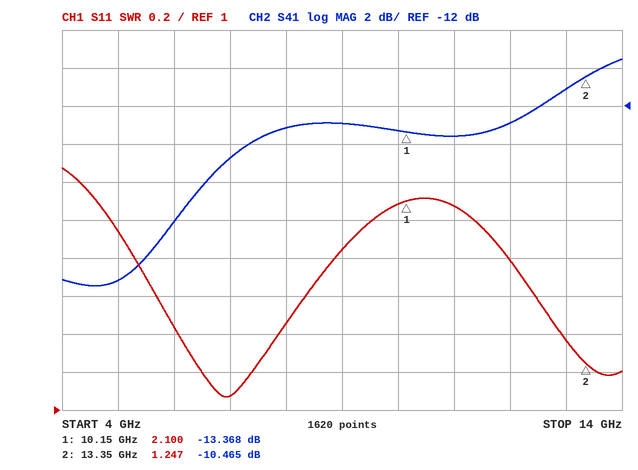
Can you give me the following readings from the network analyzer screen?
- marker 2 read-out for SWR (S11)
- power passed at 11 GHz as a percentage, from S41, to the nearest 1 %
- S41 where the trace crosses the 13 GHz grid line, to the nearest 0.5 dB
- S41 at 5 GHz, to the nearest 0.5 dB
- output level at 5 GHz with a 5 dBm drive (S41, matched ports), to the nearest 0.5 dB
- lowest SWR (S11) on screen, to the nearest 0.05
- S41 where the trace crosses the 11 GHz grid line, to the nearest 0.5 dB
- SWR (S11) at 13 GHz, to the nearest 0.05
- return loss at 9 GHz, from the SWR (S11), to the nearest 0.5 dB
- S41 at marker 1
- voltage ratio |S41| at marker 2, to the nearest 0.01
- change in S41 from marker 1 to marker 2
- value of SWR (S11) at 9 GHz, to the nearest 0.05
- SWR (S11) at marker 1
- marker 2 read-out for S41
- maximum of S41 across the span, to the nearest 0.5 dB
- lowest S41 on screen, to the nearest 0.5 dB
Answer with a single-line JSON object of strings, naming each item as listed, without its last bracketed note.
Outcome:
{"marker 2 read-out for SWR": "1.247", "power passed at 11 GHz as a percentage, from S41, to the nearest 1 %": "4 %", "S41 where the trace crosses the 13 GHz grid line, to the nearest 0.5 dB": "-11.0 dB", "S41 at 5 GHz, to the nearest 0.5 dB": "-21.0 dB", "output level at 5 GHz with a 5 dBm drive (S41, matched ports), to the nearest 0.5 dB": "-16.0 dBm", "lowest SWR (S11) on screen, to the nearest 0.05": "1.05", "S41 where the trace crosses the 11 GHz grid line, to the nearest 0.5 dB": "-13.5 dB", "SWR (S11) at 13 GHz, to the nearest 0.05": "1.35", "return loss at 9 GHz, from the SWR (S11), to the nearest 0.5 dB": "10.5 dB", "S41 at marker 1": "-13.368 dB", "voltage ratio |S41| at marker 2, to the nearest 0.01": "0.30", "change in S41 from marker 1 to marker 2": "2.903 dB", "value of SWR (S11) at 9 GHz, to the nearest 0.05": "1.85", "SWR (S11) at marker 1": "2.100", "marker 2 read-out for S41": "-10.465 dB", "maximum of S41 across the span, to the nearest 0.5 dB": "-9.5 dB", "lowest S41 on screen, to the nearest 0.5 dB": "-21.5 dB"}
